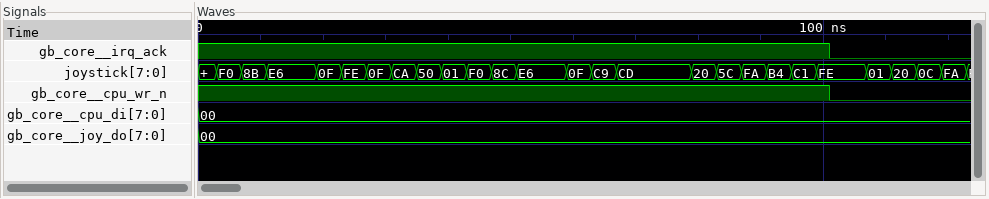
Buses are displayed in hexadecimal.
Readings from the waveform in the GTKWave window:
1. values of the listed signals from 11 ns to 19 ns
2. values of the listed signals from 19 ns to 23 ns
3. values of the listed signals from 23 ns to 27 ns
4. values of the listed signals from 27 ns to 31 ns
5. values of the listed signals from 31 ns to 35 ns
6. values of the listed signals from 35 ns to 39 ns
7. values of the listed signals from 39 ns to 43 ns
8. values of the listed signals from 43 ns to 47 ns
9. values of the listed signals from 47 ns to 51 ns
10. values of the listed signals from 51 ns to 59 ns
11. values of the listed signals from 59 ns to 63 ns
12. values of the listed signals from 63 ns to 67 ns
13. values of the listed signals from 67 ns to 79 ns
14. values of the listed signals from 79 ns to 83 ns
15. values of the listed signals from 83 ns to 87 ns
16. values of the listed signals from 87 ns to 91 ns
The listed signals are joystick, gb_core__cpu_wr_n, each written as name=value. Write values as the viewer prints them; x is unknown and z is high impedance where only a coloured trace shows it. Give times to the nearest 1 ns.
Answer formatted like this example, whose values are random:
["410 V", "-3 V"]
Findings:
["joystick=E6, gb_core__cpu_wr_n=1", "joystick=0F, gb_core__cpu_wr_n=1", "joystick=FE, gb_core__cpu_wr_n=1", "joystick=0F, gb_core__cpu_wr_n=1", "joystick=CA, gb_core__cpu_wr_n=1", "joystick=50, gb_core__cpu_wr_n=1", "joystick=01, gb_core__cpu_wr_n=1", "joystick=F0, gb_core__cpu_wr_n=1", "joystick=8C, gb_core__cpu_wr_n=1", "joystick=E6, gb_core__cpu_wr_n=1", "joystick=0F, gb_core__cpu_wr_n=1", "joystick=C9, gb_core__cpu_wr_n=1", "joystick=CD, gb_core__cpu_wr_n=1", "joystick=20, gb_core__cpu_wr_n=1", "joystick=5C, gb_core__cpu_wr_n=1", "joystick=FA, gb_core__cpu_wr_n=1"]
